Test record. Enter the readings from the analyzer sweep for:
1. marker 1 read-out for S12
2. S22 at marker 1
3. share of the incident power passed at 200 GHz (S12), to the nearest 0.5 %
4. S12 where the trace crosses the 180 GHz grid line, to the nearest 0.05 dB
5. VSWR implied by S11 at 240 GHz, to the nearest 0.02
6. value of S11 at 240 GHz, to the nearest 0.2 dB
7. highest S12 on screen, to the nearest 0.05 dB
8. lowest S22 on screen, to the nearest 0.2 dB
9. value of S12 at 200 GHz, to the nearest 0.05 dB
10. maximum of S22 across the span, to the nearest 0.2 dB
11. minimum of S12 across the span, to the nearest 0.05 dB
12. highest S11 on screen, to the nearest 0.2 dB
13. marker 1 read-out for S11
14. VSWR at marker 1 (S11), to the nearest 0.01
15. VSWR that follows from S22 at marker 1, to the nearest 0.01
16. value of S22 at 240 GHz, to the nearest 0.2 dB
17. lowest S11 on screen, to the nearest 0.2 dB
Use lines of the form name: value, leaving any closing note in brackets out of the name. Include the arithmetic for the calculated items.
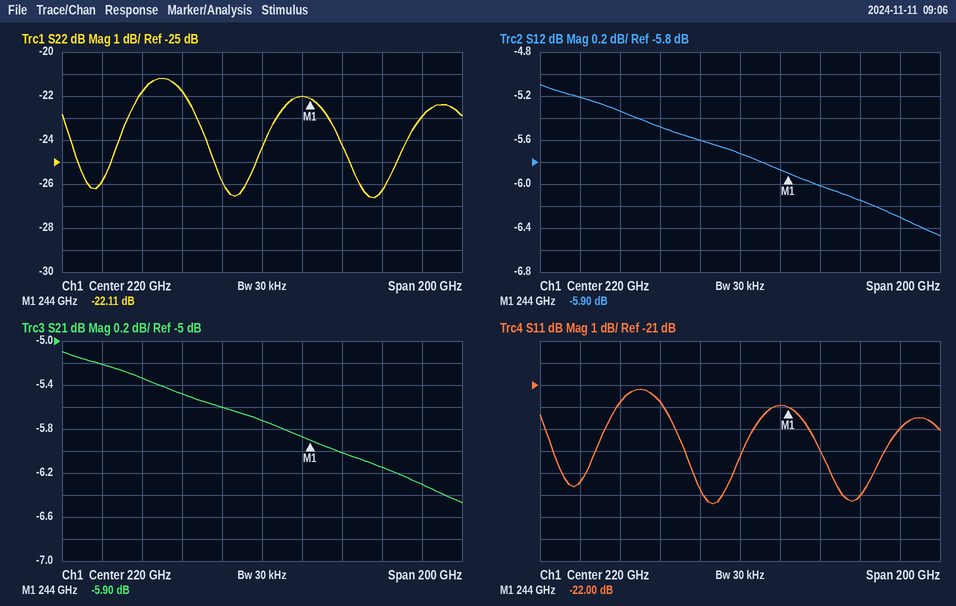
marker 1 read-out for S12: -5.90 dB
S22 at marker 1: -22.11 dB
share of the incident power passed at 200 GHz (S12), to the nearest 0.5 %: 10^(-5.6/10) ≈ 27.5 %
S12 where the trace crosses the 180 GHz grid line, to the nearest 0.05 dB: -5.50 dB
VSWR implied by S11 at 240 GHz, to the nearest 0.02: |Γ| = 10^(-22/20) = 0.0794; VSWR = (1 + 0.0794)/(1 − 0.0794) ≈ 1.17, so 1.18 to the nearest 0.02
value of S11 at 240 GHz, to the nearest 0.2 dB: -22.0 dB
highest S12 on screen, to the nearest 0.05 dB: -5.10 dB
lowest S22 on screen, to the nearest 0.2 dB: -26.6 dB
value of S12 at 200 GHz, to the nearest 0.05 dB: -5.60 dB
maximum of S22 across the span, to the nearest 0.2 dB: -21.2 dB
minimum of S12 across the span, to the nearest 0.05 dB: -6.45 dB
highest S11 on screen, to the nearest 0.2 dB: -21.2 dB
marker 1 read-out for S11: -22.00 dB
VSWR at marker 1 (S11), to the nearest 0.01: (1 + 0.0794)/(1 − 0.0794) ≈ 1.17
VSWR that follows from S22 at marker 1, to the nearest 0.01: (1 + 0.0784)/(1 − 0.0784) ≈ 1.17
value of S22 at 240 GHz, to the nearest 0.2 dB: -22.0 dB
lowest S11 on screen, to the nearest 0.2 dB: -26.4 dB
